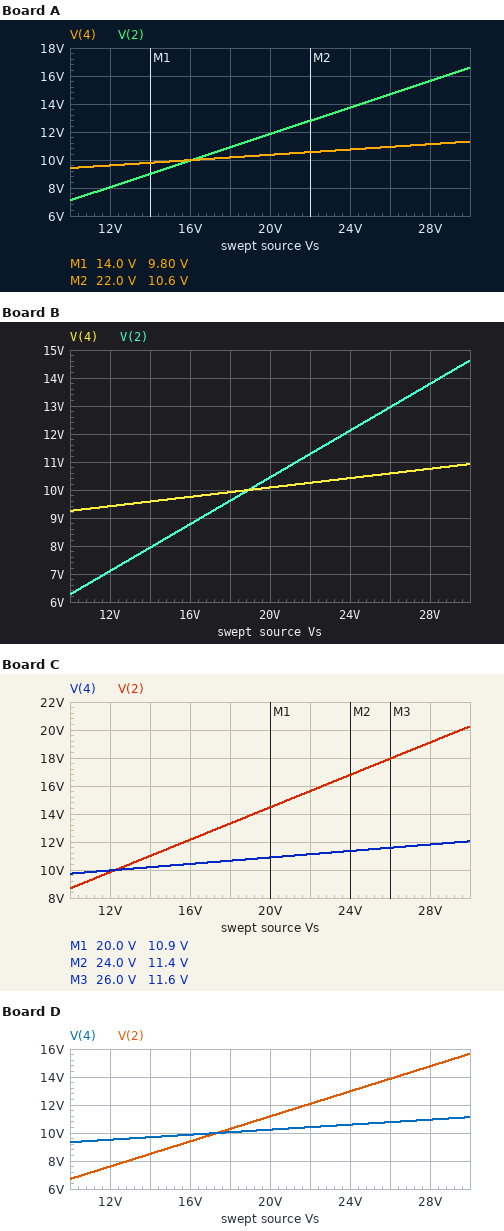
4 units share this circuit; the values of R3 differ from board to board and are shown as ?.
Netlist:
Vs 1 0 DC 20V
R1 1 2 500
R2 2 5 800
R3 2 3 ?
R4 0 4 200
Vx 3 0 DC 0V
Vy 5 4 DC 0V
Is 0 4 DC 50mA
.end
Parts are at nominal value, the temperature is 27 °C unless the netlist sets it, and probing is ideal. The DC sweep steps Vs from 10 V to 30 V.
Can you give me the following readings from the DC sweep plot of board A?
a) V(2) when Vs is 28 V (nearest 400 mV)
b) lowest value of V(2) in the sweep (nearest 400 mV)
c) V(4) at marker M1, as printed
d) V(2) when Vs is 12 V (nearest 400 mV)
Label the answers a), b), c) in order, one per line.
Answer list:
a) 15.6 V
b) 7.2 V
c) 9.80 V
d) 8.0 V
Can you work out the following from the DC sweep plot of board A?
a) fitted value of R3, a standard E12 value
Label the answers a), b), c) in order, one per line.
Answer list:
a) 820 Ω
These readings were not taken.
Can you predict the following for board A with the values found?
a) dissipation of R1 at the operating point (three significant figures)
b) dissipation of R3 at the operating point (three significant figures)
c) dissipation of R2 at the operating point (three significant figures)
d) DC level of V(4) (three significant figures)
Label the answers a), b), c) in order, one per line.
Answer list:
a) 133 mW
b) 171 mW
c) 2.74 mW
d) 10.4 V
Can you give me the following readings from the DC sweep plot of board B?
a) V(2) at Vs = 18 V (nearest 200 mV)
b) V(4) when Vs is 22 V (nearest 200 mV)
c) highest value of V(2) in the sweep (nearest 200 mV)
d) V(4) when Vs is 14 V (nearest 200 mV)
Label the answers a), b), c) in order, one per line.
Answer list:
a) 9.6 V
b) 10.2 V
c) 14.6 V
d) 9.6 V
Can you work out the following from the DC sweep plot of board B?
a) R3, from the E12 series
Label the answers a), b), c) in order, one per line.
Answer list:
a) 560 Ω
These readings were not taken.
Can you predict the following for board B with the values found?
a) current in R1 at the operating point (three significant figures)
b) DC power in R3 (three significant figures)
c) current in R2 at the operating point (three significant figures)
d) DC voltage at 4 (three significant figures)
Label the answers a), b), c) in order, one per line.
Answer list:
a) 19.1 mA
b) 195 mW
c) 448 µA
d) 10.1 V
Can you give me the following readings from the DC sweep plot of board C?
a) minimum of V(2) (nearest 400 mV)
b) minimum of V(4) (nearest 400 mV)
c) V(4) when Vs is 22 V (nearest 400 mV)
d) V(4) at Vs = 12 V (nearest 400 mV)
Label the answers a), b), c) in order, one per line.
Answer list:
a) 8.8 V
b) 9.6 V
c) 11.2 V
d) 10.0 V
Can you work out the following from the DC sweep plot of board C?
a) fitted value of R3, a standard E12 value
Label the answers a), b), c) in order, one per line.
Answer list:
a) 2.2 kΩ
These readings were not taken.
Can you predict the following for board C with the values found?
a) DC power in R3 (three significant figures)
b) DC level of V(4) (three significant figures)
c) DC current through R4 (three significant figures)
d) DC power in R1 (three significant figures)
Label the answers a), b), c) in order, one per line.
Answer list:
a) 95.2 mW
b) 10.9 V
c) 54.5 mA
d) 61.1 mW
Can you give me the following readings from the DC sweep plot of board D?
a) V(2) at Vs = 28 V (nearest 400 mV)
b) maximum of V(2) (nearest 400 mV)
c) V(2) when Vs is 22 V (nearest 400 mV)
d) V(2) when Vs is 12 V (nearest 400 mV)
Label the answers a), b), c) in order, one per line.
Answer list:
a) 14.8 V
b) 15.6 V
c) 12.0 V
d) 7.6 V
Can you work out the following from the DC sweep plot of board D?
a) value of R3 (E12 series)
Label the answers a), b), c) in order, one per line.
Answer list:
a) 680 Ω
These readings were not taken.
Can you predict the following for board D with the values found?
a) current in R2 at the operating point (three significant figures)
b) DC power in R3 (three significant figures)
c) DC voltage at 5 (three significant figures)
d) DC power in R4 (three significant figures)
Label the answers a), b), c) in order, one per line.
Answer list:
a) 1.18 mA
b) 184 mW
c) 10.2 V
d) 524 mW
